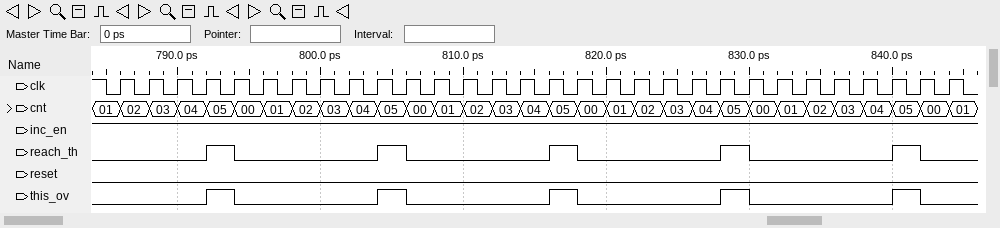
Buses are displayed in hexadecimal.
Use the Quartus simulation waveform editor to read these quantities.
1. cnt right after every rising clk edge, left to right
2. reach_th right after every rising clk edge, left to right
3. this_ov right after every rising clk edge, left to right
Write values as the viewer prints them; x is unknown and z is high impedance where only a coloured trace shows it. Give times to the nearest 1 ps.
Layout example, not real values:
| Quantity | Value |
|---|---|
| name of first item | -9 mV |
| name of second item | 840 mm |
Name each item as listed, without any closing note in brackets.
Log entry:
| Quantity | Value |
|---|---|
| cnt right after every rising clk edge, left to right | 02, 03, 04, 05, 00, 01, 02, 03, 04, 05, 00, 01, 02, 03, 04, 05, 00, 01, 02, 03, 04, 05, 00, 01, 02, 03, 04, 05, 00, 01 |
| reach_th right after every rising clk edge, left to right | 0 0 0 1 0 0 0 0 0 1 0 0 0 0 0 1 0 0 0 0 0 1 0 0 0 0 0 1 0 0 |
| this_ov right after every rising clk edge, left to right | 0 0 0 1 0 0 0 0 0 1 0 0 0 0 0 1 0 0 0 0 0 1 0 0 0 0 0 1 0 0 |
